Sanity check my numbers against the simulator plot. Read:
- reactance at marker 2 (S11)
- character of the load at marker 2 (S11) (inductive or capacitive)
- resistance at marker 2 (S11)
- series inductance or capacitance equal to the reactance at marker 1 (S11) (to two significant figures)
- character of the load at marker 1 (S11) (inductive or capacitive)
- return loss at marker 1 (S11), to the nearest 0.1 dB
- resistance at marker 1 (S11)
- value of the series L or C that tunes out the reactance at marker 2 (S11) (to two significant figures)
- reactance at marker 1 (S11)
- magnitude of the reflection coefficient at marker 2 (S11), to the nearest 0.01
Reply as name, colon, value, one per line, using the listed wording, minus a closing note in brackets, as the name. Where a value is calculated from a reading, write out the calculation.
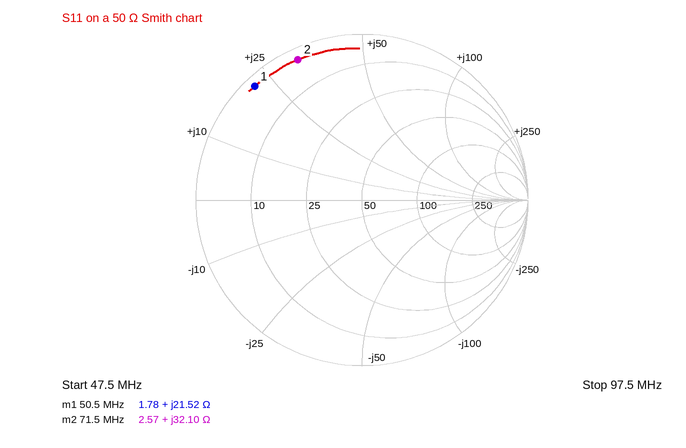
reactance at marker 2: +32.10 Ω
character of the load at marker 2 (S11): inductive
resistance at marker 2: 2.57 Ω
series inductance or capacitance equal to the reactance at marker 1 (S11): L = 21.52 Ω/(2π × 50.5 MHz) ≈ 68 nH
character of the load at marker 1 (S11): inductive
return loss at marker 1 (S11), to the nearest 0.1 dB: 0.5 dB
resistance at marker 1: 1.78 Ω
value of the series L or C that tunes out the reactance at marker 2 (S11): C = 1/(2π × 71.5 MHz × 32.1 Ω) ≈ 69 pF
reactance at marker 1: +21.52 Ω
magnitude of the reflection coefficient at marker 2 (S11), to the nearest 0.01: 0.93
